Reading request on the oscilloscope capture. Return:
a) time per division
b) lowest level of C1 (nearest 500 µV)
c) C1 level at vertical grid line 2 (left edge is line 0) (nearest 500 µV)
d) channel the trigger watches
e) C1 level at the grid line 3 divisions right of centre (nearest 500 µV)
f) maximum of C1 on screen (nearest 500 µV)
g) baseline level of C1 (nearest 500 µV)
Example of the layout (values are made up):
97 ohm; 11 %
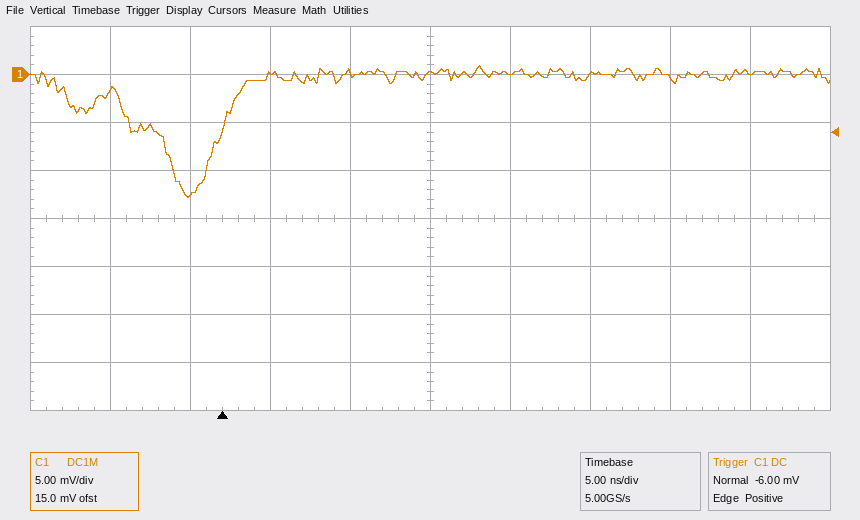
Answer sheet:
5 ns; -13.0 mV; -12.5 mV; C1; -500 µV; 1.0 mV; 0.0 mV
